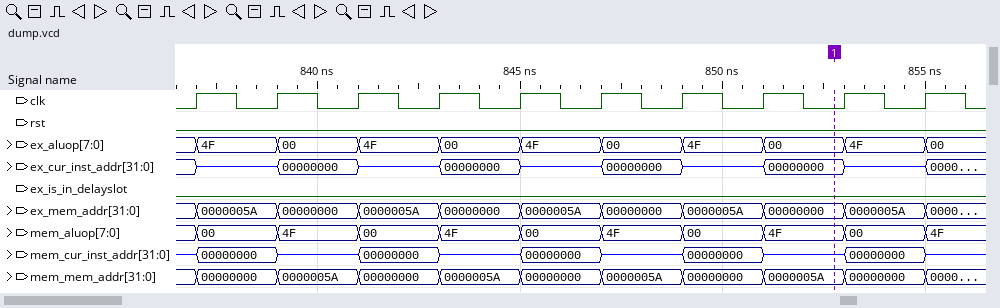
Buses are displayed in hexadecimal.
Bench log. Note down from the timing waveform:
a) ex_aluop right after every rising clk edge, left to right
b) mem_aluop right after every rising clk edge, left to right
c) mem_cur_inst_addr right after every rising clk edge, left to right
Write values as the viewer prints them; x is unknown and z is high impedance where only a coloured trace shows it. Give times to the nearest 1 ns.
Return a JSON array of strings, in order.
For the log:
["4F, 00, 4F, 00, 4F, 00, 4F, 00, 4F, 00", "00, 4F, 00, 4F, 00, 4F, 00, 4F, 00, 4F", "00000000, z, 00000000, z, 00000000, z, 00000000, z, 00000000, z"]
